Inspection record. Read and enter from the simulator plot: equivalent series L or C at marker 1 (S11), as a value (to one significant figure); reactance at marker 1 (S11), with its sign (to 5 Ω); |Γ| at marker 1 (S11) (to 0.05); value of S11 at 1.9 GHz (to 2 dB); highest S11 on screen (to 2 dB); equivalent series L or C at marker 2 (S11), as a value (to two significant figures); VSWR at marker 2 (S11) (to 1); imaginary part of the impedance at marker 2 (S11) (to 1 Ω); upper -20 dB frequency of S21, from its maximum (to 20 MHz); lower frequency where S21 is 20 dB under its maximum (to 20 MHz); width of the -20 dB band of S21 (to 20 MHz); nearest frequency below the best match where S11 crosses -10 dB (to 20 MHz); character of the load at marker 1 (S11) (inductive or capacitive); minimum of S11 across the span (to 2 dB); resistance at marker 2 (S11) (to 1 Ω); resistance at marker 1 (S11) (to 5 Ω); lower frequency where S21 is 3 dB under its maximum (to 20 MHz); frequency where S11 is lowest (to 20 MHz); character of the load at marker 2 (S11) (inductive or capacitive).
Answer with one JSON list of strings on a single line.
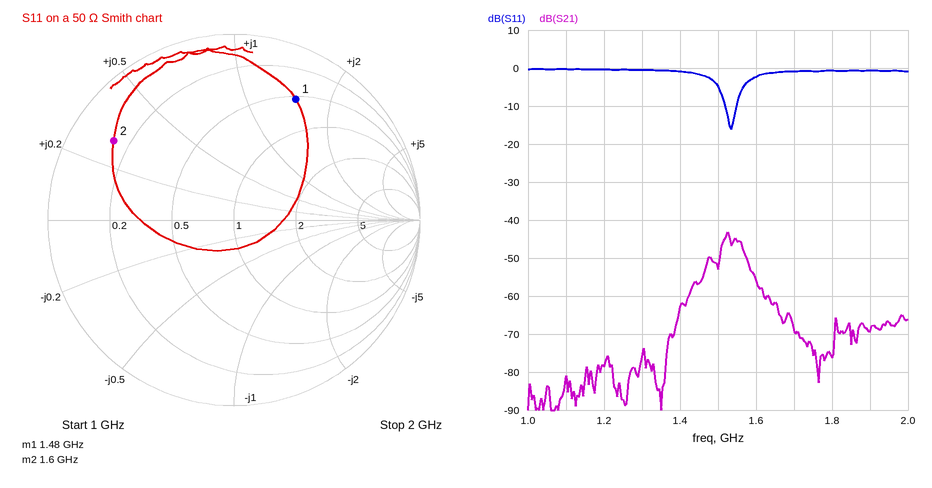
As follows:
["8 nH", "+75 Ω", "0.75", "0 dB", "0 dB", "1.5 nH", "8", "+15 Ω", "1.66 GHz", "1.40 GHz", "260 MHz", "1.52 GHz", "inductive", "-16 dB", "7 Ω", "25 Ω", "1.52 GHz", "1.54 GHz", "inductive"]
